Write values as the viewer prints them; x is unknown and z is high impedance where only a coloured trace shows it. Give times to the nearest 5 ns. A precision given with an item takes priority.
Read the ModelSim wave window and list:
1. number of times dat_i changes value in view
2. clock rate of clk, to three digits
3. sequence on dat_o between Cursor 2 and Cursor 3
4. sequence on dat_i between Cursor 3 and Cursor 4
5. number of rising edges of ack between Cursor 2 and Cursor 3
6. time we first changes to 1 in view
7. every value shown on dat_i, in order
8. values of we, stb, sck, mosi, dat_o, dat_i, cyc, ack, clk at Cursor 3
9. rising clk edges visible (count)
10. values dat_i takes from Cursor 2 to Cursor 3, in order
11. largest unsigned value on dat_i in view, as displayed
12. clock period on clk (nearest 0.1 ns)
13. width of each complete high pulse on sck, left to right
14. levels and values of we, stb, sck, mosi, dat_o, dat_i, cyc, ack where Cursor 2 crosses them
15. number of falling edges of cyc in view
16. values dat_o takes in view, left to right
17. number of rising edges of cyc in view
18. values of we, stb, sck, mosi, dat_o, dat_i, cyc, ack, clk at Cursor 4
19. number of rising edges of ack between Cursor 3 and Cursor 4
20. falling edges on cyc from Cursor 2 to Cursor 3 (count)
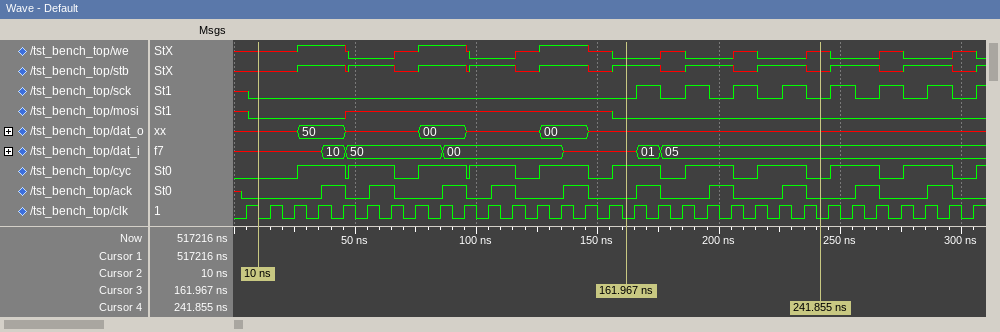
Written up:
6
100 MHz
x, 50, x, 00, x, 00, x
x, 01, 05
5
25 ns
x, 10, 50, 00, x, 01, 05
we=0, stb=1, sck=0, mosi=0, dat_o=x, dat_i=x, cyc=1, ack=0, clk=0
31
x, 10, 50, 00, x
50
10 ns
10 ns, 10 ns, 10 ns, 10 ns, 10 ns, 10 ns, 10 ns
we=x, stb=x, sck=0, mosi=0, dat_o=x, dat_i=x, cyc=0, ack=0
10
x, 50, x, 00, x, 00, x
11
we=x, stb=x, sck=0, mosi=0, dat_o=x, dat_i=05, cyc=0, ack=0, clk=0
3
5
